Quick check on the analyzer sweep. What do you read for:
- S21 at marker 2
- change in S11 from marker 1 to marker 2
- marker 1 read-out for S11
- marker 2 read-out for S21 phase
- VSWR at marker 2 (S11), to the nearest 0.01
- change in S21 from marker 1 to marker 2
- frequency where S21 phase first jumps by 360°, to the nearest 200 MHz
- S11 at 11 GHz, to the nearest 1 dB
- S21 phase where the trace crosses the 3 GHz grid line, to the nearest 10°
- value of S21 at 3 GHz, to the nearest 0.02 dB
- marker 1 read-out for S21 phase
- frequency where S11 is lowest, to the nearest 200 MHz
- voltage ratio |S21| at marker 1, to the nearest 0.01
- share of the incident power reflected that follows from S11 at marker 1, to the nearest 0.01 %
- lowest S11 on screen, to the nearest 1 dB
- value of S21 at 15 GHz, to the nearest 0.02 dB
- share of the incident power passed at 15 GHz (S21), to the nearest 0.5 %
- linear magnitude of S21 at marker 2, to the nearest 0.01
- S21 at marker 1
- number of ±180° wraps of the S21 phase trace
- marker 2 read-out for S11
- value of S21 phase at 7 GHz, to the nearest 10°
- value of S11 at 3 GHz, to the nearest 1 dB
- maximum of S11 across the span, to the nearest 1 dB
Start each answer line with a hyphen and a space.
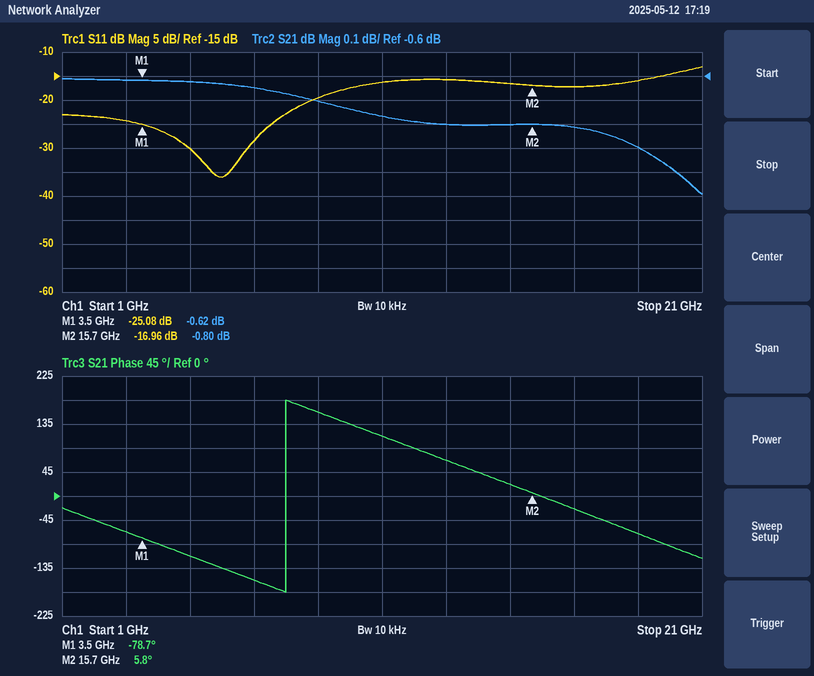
- -0.80 dB
- 8.12 dB
- -25.08 dB
- 5.8°
- 1.33
- -0.18 dB
- 8.0 GHz
- -16 dB
- -70°
- -0.62 dB
- -78.7°
- 6.0 GHz
- 0.93
- 0.31 %
- -36 dB
- -0.80 dB
- 83.0 %
- 0.91
- -0.62 dB
- 1
- -16.96 dB
- -160°
- -24 dB
- -13 dB
